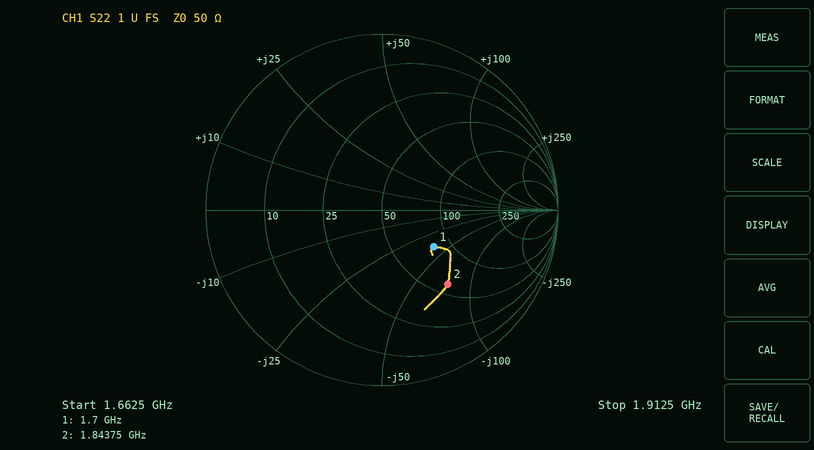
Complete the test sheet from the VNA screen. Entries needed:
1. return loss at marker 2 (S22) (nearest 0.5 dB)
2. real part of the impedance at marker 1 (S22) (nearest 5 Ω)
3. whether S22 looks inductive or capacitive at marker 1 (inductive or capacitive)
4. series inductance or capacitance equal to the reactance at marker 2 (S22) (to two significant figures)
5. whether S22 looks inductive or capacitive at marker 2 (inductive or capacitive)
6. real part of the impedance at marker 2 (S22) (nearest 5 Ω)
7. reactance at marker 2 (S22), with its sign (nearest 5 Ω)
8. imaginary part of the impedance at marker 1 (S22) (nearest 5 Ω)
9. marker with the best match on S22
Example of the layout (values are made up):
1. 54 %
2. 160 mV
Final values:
1. 5.0 dB
2. 80 Ω
3. capacitive
4. 1.2 pF
5. capacitive
6. 60 Ω
7. -75 Ω
8. -40 Ω
9. marker 1
